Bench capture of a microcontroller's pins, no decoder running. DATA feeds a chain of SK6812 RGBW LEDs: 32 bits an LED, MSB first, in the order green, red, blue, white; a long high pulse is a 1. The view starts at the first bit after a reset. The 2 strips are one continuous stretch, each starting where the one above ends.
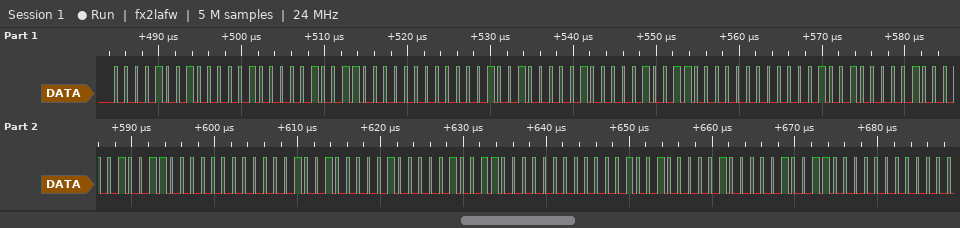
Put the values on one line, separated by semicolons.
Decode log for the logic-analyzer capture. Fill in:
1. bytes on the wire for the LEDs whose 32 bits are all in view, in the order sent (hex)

09 04 13 00 09 04 13 00 09 04 13 00 09 04 13 00 09 04 13 00
